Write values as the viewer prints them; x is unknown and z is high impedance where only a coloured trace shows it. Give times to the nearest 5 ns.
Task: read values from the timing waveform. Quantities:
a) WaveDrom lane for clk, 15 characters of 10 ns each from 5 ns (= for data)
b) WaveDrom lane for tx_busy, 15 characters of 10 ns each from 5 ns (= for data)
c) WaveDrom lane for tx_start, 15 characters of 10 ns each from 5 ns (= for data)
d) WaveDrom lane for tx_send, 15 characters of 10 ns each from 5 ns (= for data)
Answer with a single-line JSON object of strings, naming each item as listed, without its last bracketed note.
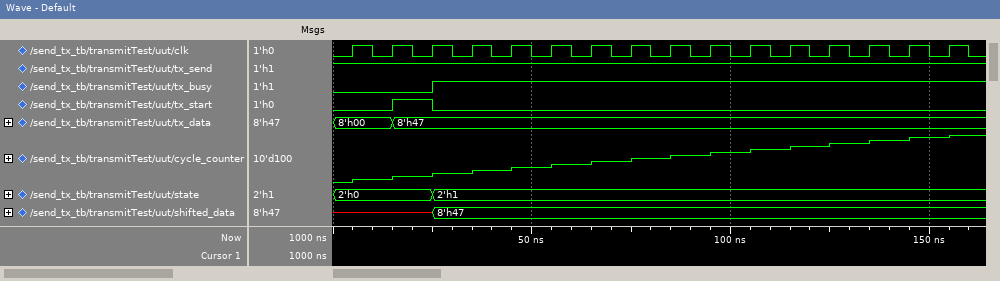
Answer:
{"WaveDrom lane for clk, 15 characters of 10 ns each from 5 ns": "{name: 'clk', wave: 'p..............'}", "WaveDrom lane for tx_busy, 15 characters of 10 ns each from 5 ns": "{name: 'tx_busy', wave: '0.1............'}", "WaveDrom lane for tx_start, 15 characters of 10 ns each from 5 ns": "{name: 'tx_start', wave: '010............'}", "WaveDrom lane for tx_send, 15 characters of 10 ns each from 5 ns": "{name: 'tx_send', wave: '1..............'}"}
